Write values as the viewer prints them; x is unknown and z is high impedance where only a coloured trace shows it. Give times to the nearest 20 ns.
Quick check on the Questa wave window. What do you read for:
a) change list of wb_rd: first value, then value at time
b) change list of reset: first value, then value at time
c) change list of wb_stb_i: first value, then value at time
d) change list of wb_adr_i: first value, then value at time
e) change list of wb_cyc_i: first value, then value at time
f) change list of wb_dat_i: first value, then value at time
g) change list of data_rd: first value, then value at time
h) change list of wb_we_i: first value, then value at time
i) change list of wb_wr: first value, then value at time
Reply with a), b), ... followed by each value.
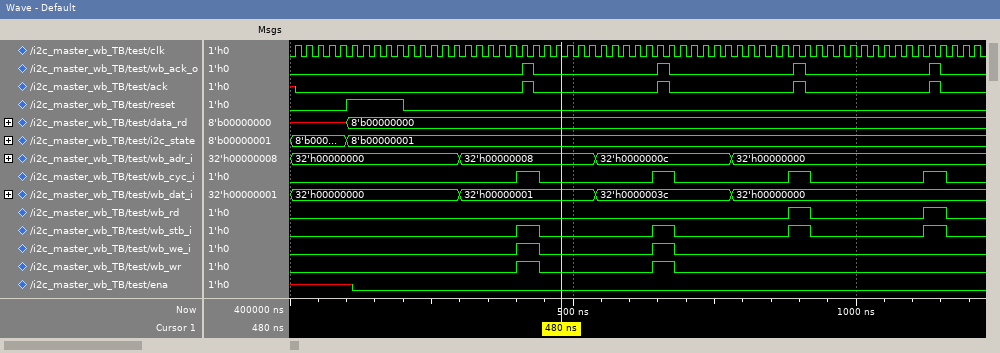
a) 0, 1 at 880 ns, 0 at 920 ns, 1 at 1120 ns, 0 at 1160 ns
b) 0, 1 at 100 ns, 0 at 200 ns
c) 0, 1 at 400 ns, 0 at 440 ns, 1 at 640 ns, 0 at 680 ns, 1 at 880 ns, 0 at 920 ns, 1 at 1120 ns, 0 at 1160 ns
d) 32'h00000000, 32'h00000008 at 300 ns, 32'h0000000c at 540 ns, 32'h00000000 at 780 ns
e) 0, 1 at 400 ns, 0 at 440 ns, 1 at 640 ns, 0 at 680 ns, 1 at 880 ns, 0 at 920 ns, 1 at 1120 ns, 0 at 1160 ns
f) 32'h00000000, 32'h00000001 at 300 ns, 32'h0000003c at 540 ns, 32'h00000000 at 780 ns
g) x, 8'b00000000 at 100 ns
h) 0, 1 at 400 ns, 0 at 440 ns, 1 at 640 ns, 0 at 680 ns
i) 0, 1 at 400 ns, 0 at 440 ns, 1 at 640 ns, 0 at 680 ns
